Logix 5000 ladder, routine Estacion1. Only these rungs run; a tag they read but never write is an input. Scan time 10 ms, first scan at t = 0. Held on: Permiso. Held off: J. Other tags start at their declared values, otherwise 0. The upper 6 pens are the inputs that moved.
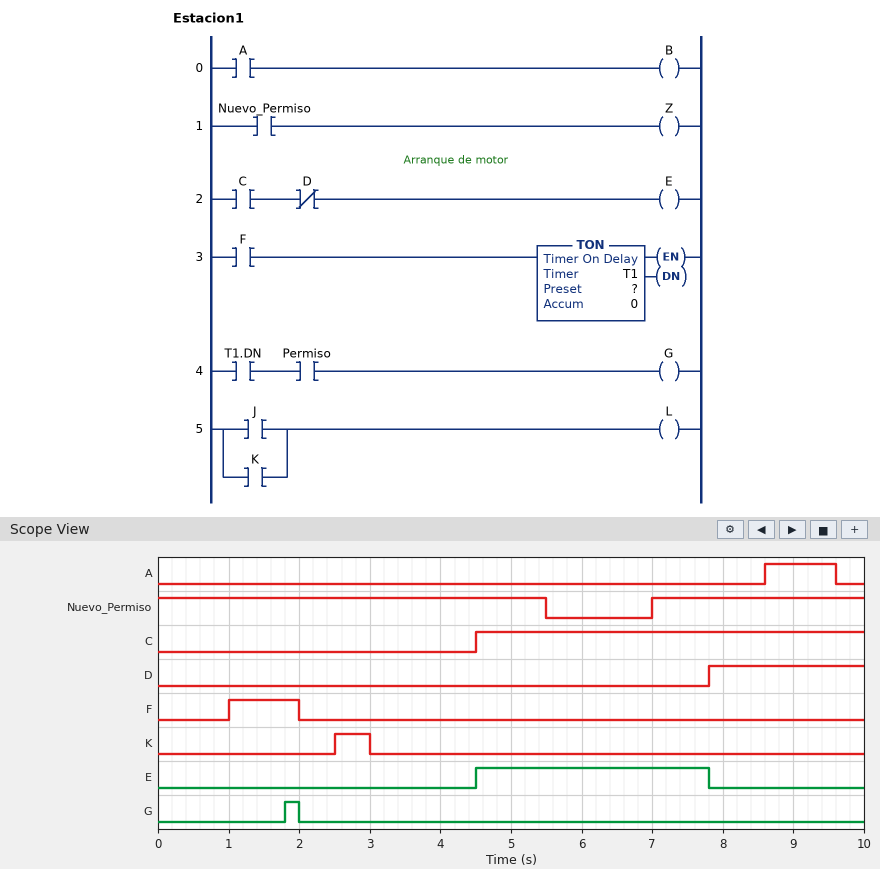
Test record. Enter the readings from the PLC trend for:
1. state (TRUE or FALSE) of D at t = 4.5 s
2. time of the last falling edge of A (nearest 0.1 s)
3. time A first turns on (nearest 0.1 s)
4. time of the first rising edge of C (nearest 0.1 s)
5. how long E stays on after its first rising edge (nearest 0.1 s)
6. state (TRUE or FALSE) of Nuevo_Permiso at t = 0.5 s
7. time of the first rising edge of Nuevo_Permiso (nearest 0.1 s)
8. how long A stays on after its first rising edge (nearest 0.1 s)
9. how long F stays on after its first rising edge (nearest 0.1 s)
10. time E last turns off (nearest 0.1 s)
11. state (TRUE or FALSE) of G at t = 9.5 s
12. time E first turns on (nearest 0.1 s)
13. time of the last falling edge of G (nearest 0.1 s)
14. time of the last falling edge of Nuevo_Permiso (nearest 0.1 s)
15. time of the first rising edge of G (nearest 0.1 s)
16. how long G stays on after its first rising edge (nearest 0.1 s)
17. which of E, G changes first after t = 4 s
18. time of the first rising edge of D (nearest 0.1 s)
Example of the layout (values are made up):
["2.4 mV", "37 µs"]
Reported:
["FALSE", "9.6 s", "8.6 s", "4.5 s", "3.3 s", "TRUE", "7.0 s", "1.0 s", "1.0 s", "7.8 s", "FALSE", "4.5 s", "2.0 s", "5.5 s", "1.8 s", "0.2 s", "E", "7.8 s"]
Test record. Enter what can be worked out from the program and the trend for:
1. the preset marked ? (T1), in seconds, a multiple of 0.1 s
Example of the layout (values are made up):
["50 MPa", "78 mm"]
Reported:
["0.8 s"]
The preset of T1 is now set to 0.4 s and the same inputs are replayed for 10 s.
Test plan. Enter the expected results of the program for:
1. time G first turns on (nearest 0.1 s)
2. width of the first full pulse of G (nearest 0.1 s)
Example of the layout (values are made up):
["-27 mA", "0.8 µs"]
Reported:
["1.4 s", "0.6 s"]
